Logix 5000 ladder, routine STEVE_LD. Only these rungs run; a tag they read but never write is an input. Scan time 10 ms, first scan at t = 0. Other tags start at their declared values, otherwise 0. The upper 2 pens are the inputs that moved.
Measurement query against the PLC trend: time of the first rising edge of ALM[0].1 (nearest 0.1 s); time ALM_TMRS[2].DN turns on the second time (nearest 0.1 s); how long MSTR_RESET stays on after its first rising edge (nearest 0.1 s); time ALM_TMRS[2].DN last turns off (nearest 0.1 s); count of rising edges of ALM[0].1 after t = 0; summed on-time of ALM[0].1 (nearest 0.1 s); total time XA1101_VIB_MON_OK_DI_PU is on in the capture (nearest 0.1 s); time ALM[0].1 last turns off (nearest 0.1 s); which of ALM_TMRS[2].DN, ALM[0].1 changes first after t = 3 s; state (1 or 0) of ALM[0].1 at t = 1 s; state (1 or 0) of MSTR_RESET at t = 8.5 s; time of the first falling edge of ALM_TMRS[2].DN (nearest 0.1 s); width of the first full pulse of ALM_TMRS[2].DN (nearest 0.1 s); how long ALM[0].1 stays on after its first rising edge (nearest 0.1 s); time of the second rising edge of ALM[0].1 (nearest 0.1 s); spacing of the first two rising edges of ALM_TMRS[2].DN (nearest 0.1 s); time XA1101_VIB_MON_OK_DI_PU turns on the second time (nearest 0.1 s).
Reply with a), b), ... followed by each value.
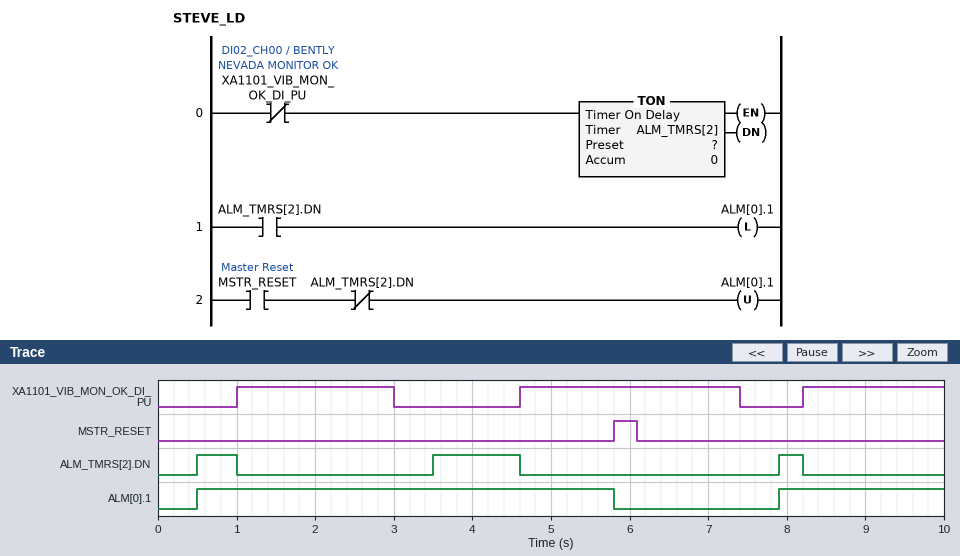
a) 0.5 s
b) 3.5 s
c) 0.3 s
d) 8.2 s
e) 2
f) 7.4 s
g) 6.6 s
h) 5.8 s
i) ALM_TMRS[2].DN
j) 1
k) 0
l) 1.0 s
m) 0.5 s
n) 5.3 s
o) 7.9 s
p) 3.0 s
q) 4.6 s
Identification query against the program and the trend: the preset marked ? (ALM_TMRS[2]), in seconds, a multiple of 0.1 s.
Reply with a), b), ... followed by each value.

a) 0.5 s
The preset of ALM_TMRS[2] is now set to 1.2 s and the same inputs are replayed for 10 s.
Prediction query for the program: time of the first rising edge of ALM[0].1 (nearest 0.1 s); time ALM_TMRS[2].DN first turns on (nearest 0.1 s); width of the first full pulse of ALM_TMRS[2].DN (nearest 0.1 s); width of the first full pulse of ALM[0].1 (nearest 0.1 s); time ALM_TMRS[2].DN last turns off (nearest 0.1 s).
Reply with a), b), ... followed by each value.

a) 4.2 s
b) 4.2 s
c) 0.4 s
d) 1.6 s
e) 4.6 s
